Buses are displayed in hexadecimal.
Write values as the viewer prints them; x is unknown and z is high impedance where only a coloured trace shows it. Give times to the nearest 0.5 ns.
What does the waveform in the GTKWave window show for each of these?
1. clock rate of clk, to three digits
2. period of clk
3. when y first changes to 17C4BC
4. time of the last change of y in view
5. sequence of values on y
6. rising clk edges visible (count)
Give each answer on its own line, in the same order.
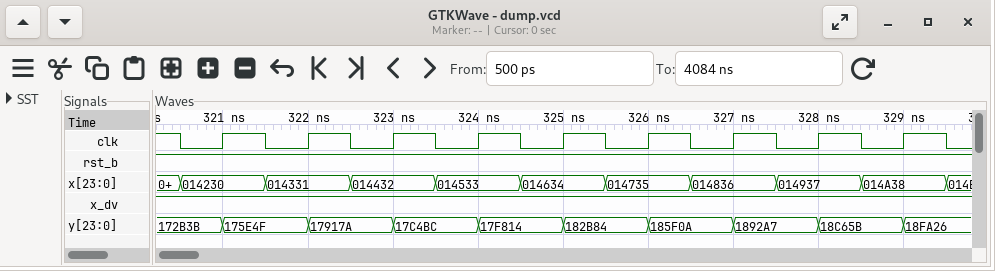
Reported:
1.00 GHz
1 ns
323 ns
329 ns
172B3B, 175E4F, 17917A, 17C4BC, 17F814, 182B84, 185F0A, 1892A7, 18C65B, 18FA26
9
